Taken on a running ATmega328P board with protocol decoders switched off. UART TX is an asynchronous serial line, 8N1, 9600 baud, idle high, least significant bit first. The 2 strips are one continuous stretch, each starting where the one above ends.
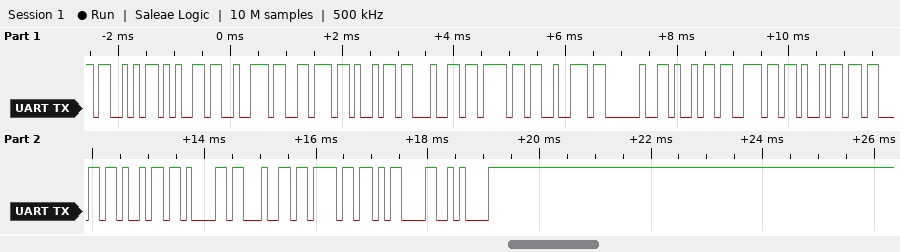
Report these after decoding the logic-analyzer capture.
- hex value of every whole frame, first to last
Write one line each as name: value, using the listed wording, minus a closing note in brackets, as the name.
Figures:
hex value of every whole frame, first to last: 0x53 0x65 0x72 0x76 0x69 0x64 0x6F 0x72 0x20 0x69 0x6E 0x69 0x63 0x69 0x61 0x64 0x6F 0x0D 0x0A
